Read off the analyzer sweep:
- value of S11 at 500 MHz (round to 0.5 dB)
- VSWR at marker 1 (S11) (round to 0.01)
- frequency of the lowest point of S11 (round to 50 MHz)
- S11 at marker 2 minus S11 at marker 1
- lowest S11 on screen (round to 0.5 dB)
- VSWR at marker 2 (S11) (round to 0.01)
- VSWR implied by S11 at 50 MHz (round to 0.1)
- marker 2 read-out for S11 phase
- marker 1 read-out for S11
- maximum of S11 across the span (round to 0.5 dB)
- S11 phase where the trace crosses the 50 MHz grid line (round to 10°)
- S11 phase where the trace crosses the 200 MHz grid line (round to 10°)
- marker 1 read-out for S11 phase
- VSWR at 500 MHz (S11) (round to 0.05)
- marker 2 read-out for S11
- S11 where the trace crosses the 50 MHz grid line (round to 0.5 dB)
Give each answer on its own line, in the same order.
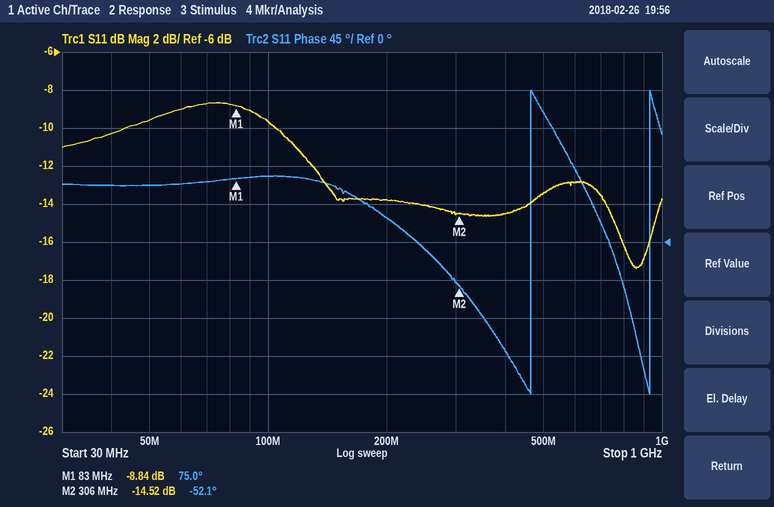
-13.5 dB
2.13
850 MHz
-5.68 dB
-17.5 dB
1.46
2.0
-52.1°
-8.84 dB
-8.5 dB
70°
30°
75.0°
1.55
-14.52 dB
-9.5 dB
